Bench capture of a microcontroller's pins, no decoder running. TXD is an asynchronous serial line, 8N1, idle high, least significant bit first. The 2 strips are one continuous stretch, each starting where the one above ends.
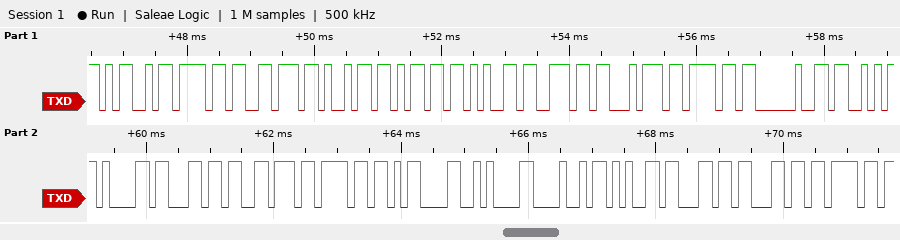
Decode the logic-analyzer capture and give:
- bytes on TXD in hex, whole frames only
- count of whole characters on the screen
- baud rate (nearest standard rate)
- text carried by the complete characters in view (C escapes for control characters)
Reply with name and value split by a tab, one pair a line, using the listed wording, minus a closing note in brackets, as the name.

bytes on TXD in hex, whole frames only	0x4D 0x6F 0x76 0x69 0x6D 0x65 0x6E 0x74 0x6F 0x20 0x53 0x61 0x6C 0x76 0x6F 0x0D 0x0A 0x48 0x65 0x6C 0x6C 0x6F
count of whole characters on the screen	22
baud rate	9600 baud
text carried by the complete characters in view	"Movimento Salvo\r\nHello"
